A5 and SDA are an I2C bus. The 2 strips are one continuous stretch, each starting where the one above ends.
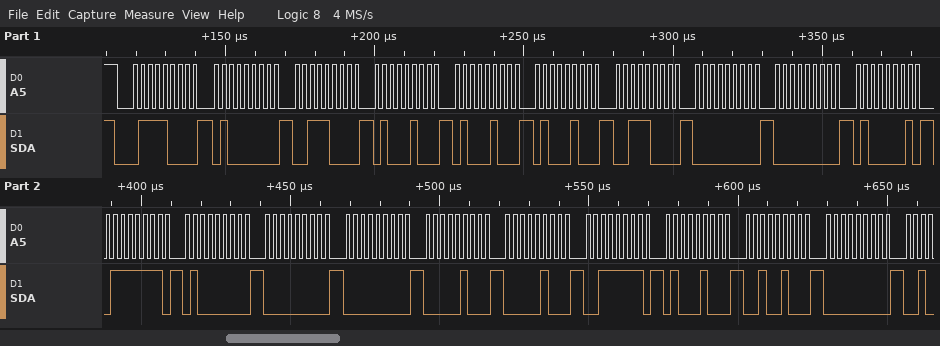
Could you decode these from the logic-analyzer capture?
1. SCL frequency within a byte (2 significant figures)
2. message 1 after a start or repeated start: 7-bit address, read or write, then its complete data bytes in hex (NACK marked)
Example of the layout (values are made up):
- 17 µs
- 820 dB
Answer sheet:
- 400 kHz
- 0x3C write: 40 38 44 44 44 38 00 00 41 7F 40 00 00 04 04 3F 44 24 00
